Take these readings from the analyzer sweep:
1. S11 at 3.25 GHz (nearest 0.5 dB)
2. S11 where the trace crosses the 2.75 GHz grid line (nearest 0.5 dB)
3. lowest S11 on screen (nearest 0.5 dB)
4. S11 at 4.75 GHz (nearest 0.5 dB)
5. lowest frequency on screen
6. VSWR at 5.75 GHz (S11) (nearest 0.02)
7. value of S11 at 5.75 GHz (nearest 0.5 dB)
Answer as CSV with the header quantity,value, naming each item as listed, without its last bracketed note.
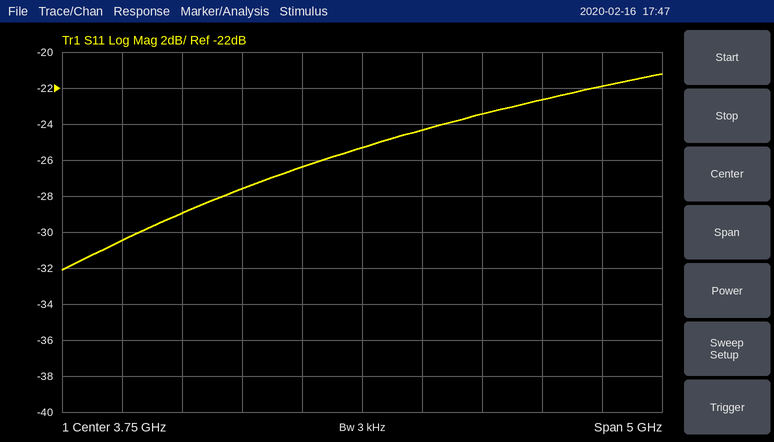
quantity,value
S11 at 3.25 GHz,-26.5 dB
S11 where the trace crosses the 2.75 GHz grid line,-27.5 dB
lowest S11 on screen,-32.0 dB
S11 at 4.75 GHz,-23.5 dB
lowest frequency on screen,1.25 GHz
VSWR at 5.75 GHz (S11),1.18
value of S11 at 5.75 GHz,-22.0 dB
